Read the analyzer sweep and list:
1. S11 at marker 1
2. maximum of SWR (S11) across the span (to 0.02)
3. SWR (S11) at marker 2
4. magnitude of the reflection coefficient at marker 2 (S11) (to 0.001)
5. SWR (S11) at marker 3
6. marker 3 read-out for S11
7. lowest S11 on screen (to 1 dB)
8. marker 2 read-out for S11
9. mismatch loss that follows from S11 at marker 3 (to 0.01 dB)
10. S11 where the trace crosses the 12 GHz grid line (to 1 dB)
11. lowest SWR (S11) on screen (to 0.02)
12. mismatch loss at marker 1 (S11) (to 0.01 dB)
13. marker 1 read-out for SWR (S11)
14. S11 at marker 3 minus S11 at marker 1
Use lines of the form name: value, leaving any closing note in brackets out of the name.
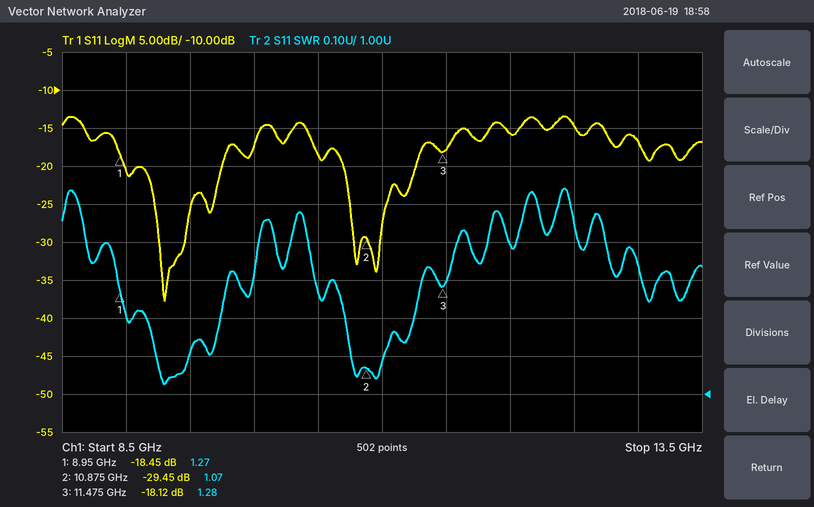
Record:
S11 at marker 1: -18.45 dB
maximum of SWR (S11) across the span: 1.54
SWR (S11) at marker 2: 1.07
magnitude of the reflection coefficient at marker 2 (S11): 0.034
SWR (S11) at marker 3: 1.28
marker 3 read-out for S11: -18.12 dB
lowest S11 on screen: -38 dB
marker 2 read-out for S11: -29.45 dB
mismatch loss that follows from S11 at marker 3: 0.07 dB
S11 where the trace crosses the 12 GHz grid line: -16 dB
lowest SWR (S11) on screen: 1.02
mismatch loss at marker 1 (S11): 0.06 dB
marker 1 read-out for SWR: 1.27
S11 at marker 3 minus S11 at marker 1: 0.33 dB
